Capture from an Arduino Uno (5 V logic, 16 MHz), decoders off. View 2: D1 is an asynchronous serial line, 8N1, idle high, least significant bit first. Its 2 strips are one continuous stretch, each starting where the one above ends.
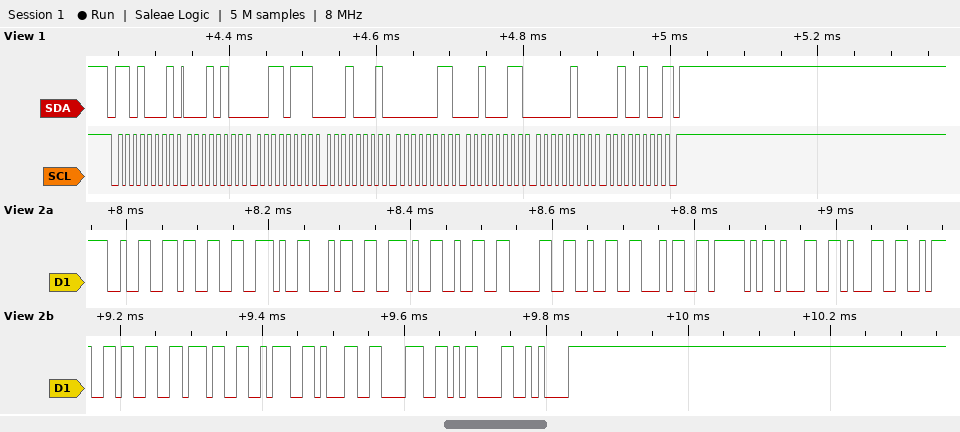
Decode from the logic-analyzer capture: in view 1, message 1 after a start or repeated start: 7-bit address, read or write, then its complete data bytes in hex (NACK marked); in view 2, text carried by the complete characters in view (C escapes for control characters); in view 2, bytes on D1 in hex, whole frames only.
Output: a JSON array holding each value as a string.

["0x68 read: 14 37 11 03 23 04 24 NACK", "\"23.4.2024_11:37:18\\r\\n\"", "32 33 2E 34 2E 32 30 32 34 5F 31 31 3A 33 37 3A 31 38 0D 0A"]
